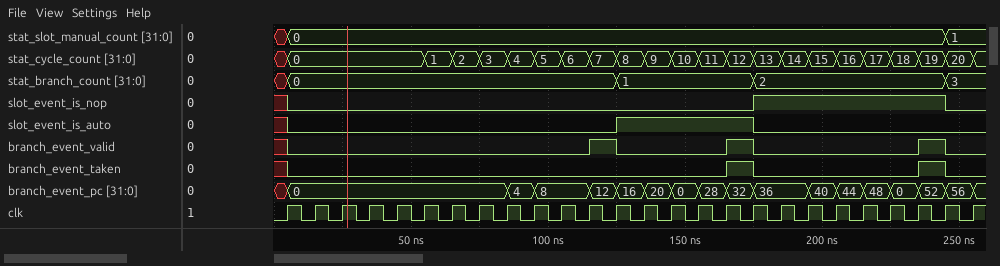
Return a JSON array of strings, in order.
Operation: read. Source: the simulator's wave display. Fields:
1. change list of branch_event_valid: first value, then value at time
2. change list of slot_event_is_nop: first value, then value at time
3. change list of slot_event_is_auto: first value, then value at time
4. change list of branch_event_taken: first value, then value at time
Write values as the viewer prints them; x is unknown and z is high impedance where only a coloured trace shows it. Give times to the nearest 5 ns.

["x, 0 at 5 ns, 1 at 115 ns, 0 at 125 ns, 1 at 165 ns, 0 at 175 ns, 1 at 235 ns, 0 at 245 ns", "x, 0 at 5 ns, 1 at 175 ns, 0 at 245 ns", "x, 0 at 5 ns, 1 at 125 ns, 0 at 175 ns", "x, 0 at 5 ns, 1 at 165 ns, 0 at 175 ns, 1 at 235 ns, 0 at 245 ns"]
